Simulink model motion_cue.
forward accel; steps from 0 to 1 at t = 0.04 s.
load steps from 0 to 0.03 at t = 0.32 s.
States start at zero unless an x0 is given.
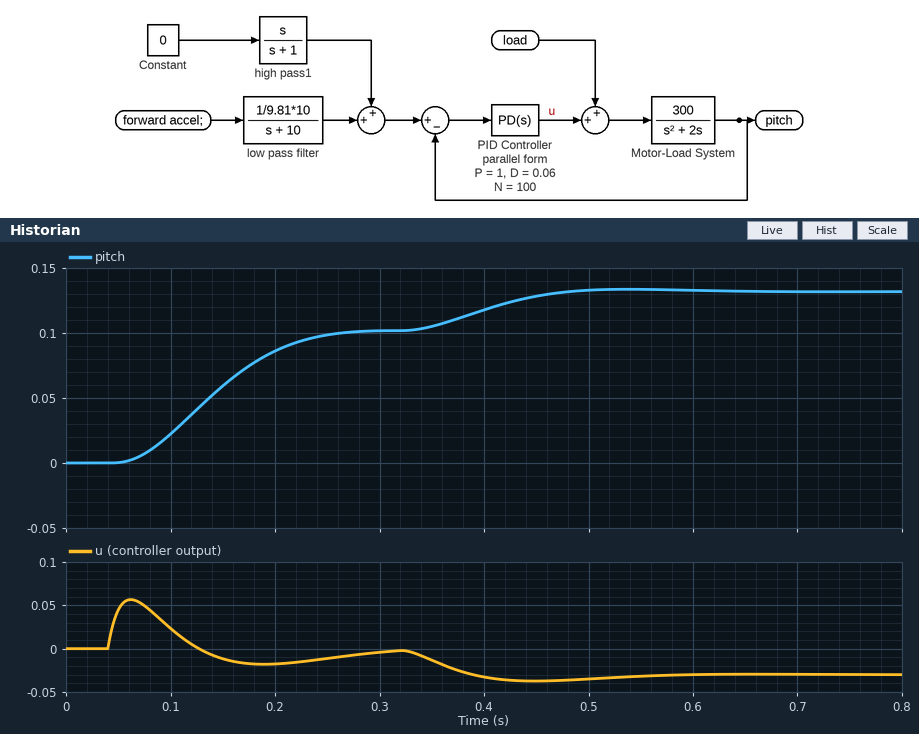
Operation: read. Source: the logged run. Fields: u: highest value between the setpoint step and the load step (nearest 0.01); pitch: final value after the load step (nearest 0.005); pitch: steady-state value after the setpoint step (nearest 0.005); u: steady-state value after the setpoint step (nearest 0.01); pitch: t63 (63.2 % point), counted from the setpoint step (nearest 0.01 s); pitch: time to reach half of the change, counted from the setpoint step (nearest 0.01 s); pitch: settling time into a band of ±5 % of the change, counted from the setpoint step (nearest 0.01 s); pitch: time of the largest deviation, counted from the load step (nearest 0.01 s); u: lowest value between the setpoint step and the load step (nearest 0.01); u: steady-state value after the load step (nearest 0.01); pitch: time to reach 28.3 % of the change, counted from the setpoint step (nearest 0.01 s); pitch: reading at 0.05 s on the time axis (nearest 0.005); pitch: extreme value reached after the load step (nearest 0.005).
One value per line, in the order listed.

0.06
0.130
0.100
0.00
0.12 s
0.10 s
0.20 s
0.22 s
-0.02
-0.03
0.07 s
0.000
0.135
